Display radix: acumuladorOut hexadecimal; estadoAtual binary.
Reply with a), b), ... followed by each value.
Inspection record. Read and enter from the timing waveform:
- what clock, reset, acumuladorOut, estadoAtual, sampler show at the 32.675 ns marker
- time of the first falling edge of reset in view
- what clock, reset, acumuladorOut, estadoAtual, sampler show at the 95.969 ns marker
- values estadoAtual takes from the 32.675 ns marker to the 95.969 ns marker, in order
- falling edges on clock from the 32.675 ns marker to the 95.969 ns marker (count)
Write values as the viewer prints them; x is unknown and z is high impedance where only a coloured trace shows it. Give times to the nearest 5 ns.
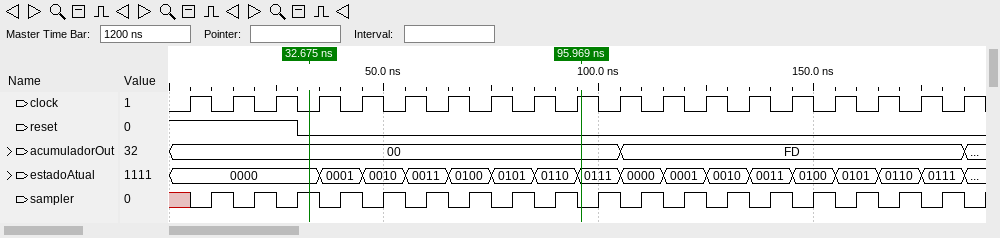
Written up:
a) clock=0, reset=0, acumuladorOut=00, estadoAtual=0000, sampler=1
b) 30 ns
c) clock=1, reset=0, acumuladorOut=00, estadoAtual=0111, sampler=0
d) 0000, 0001, 0010, 0011, 0100, 0101, 0110, 0111
e) 6
